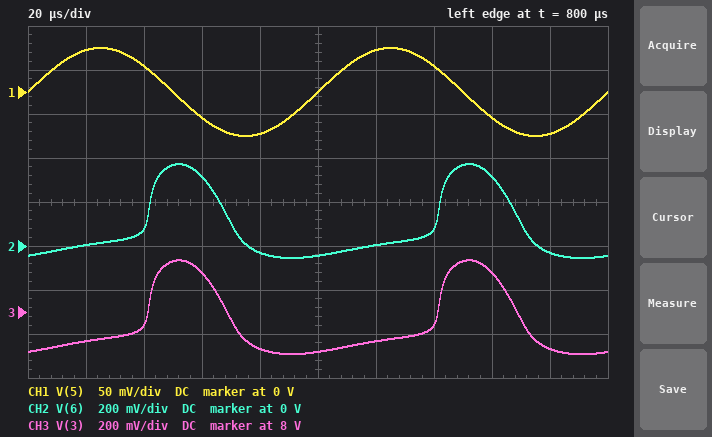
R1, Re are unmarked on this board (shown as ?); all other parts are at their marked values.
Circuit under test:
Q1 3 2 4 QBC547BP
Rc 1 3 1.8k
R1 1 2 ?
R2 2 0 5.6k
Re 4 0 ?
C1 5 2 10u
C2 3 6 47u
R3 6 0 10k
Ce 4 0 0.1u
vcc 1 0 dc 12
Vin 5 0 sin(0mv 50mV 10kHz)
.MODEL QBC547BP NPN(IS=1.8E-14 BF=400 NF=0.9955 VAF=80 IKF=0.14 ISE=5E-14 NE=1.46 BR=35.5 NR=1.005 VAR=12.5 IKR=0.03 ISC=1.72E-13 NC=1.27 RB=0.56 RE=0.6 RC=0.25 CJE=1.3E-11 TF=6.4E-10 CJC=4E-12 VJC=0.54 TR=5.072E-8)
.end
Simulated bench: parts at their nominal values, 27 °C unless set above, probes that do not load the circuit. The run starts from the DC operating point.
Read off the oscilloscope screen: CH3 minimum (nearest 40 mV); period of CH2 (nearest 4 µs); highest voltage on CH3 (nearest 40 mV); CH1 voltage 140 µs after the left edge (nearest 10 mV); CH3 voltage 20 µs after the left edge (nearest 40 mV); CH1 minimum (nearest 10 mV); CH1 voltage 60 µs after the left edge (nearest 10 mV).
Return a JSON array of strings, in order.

["7.80 V", "100 µs", "8.24 V", "30 mV", "7.88 V", "-50 mV", "-30 mV"]
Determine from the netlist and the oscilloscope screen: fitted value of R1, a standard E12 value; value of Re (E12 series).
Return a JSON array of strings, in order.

["2.2 kΩ", "3.3 kΩ"]
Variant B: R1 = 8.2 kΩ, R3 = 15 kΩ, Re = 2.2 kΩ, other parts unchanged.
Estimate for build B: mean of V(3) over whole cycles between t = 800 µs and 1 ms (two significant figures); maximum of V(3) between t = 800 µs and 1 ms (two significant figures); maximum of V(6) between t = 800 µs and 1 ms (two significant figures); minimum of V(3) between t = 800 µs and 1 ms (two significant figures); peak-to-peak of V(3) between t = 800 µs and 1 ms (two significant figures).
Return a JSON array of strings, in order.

["8.6 V", "9.1 V", "500 mV", "8.1 V", "1.0 V"]
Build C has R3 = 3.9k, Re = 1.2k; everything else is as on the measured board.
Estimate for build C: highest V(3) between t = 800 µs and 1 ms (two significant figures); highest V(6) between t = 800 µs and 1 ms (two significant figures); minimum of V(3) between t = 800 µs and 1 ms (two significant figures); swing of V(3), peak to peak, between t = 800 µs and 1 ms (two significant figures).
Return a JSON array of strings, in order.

["5.8 V", "47 mV", "5.7 V", "94 mV"]
